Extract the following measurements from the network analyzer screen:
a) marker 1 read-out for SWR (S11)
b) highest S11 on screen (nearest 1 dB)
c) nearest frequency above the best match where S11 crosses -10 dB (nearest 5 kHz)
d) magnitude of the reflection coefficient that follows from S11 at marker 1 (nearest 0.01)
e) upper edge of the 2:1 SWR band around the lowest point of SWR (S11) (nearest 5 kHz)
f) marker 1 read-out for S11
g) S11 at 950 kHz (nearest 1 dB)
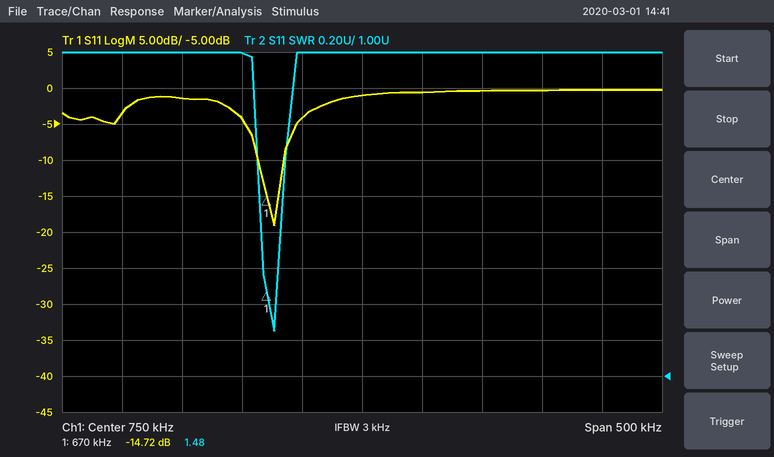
1.48
0 dB
685 kHz
0.18
685 kHz
-14.72 dB
0 dB
